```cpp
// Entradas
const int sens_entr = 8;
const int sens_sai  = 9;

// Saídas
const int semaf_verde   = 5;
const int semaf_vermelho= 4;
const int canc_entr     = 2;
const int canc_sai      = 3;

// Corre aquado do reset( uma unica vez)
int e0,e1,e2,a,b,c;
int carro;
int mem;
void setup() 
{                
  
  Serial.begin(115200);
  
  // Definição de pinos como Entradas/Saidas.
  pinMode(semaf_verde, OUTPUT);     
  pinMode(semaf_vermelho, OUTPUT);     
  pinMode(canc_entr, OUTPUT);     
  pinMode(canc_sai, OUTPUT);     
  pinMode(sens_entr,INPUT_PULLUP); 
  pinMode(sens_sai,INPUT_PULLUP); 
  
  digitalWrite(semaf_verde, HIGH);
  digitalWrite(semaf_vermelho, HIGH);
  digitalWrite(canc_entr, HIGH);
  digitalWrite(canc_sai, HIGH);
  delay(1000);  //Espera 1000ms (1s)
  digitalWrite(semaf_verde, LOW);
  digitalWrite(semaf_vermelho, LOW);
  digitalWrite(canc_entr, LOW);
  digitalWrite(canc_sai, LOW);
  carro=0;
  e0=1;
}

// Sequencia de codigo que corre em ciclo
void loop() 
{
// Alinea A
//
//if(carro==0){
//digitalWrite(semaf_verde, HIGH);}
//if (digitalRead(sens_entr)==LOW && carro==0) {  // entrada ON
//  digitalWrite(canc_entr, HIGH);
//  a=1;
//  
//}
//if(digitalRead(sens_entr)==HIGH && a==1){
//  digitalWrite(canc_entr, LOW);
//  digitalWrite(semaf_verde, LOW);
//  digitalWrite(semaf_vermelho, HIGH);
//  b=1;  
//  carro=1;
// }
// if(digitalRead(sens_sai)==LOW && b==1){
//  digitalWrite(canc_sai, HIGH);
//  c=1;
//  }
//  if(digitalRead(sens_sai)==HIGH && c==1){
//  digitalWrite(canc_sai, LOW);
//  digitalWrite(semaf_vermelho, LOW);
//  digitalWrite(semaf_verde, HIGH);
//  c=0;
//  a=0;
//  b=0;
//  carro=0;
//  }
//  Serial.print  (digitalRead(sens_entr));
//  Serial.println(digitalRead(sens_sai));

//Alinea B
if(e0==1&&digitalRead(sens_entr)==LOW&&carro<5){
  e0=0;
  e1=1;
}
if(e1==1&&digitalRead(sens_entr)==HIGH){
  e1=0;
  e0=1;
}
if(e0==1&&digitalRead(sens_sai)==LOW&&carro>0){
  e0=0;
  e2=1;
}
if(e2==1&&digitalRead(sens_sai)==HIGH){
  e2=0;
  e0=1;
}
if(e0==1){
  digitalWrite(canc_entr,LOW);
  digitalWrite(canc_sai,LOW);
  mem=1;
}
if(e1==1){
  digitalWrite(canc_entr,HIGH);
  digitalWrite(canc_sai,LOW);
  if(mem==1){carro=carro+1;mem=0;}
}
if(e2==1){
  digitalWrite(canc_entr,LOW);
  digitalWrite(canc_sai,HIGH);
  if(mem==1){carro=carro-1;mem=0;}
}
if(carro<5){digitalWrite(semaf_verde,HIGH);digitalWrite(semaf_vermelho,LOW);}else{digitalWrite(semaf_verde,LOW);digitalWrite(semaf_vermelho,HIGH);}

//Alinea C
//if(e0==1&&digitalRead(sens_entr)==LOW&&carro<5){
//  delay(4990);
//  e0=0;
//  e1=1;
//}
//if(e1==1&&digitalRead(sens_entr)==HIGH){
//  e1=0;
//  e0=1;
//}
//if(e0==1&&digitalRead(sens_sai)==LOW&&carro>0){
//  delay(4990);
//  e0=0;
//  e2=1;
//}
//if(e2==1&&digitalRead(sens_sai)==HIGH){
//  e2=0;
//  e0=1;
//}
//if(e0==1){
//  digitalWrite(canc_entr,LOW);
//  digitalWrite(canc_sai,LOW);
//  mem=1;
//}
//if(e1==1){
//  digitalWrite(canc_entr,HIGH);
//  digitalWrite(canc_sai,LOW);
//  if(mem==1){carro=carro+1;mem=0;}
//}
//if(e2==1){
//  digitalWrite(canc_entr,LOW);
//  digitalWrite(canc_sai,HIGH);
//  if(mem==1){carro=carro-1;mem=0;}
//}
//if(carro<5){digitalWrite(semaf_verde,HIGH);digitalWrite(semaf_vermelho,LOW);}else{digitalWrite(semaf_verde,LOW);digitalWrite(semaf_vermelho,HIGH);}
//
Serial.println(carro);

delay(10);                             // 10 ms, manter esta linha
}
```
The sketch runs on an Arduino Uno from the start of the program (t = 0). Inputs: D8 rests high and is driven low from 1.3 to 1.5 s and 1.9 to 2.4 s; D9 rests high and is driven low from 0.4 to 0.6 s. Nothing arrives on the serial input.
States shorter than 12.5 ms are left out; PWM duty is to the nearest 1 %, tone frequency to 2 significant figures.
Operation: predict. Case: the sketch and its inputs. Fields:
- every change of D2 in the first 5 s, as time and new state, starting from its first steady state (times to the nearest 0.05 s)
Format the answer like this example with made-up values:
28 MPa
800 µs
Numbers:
0 s high; 1 s low; 1.3 s high; 1.5 s low; 1.9 s high; 2.4 s low
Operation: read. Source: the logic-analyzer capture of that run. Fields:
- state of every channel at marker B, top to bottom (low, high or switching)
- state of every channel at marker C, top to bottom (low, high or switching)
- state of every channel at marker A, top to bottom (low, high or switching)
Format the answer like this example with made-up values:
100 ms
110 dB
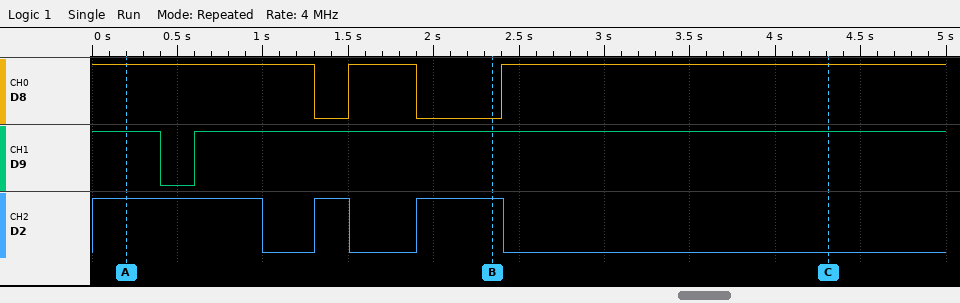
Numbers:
D8 low, D9 high, D2 high
D8 high, D9 high, D2 low
D8 high, D9 high, D2 high
